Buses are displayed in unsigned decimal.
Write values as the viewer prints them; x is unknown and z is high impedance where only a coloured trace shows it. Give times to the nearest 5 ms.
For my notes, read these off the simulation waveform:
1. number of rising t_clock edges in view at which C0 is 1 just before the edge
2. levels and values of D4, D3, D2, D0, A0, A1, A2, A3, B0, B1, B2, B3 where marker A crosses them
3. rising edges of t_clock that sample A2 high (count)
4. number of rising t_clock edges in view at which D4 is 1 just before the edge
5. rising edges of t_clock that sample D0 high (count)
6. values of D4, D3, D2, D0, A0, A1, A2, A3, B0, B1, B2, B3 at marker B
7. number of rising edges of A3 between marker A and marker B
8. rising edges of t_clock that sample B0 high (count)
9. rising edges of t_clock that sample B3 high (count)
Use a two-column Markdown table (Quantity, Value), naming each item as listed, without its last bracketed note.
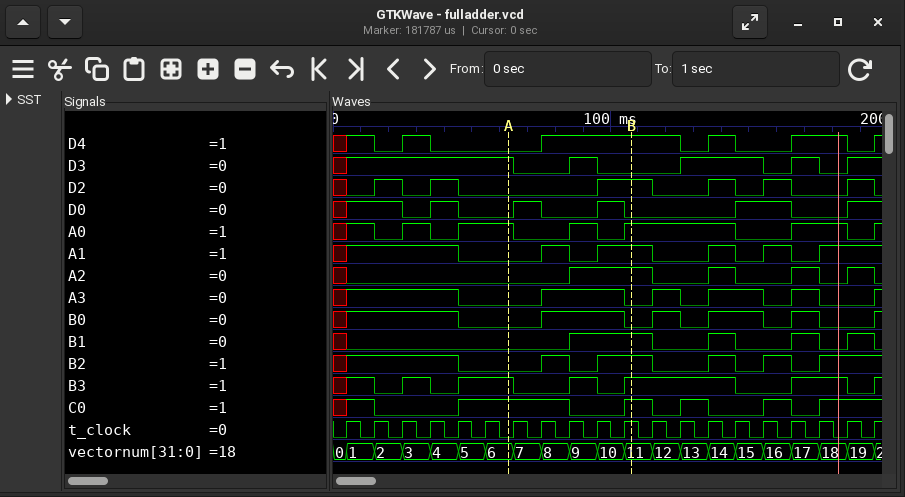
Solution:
| Quantity | Value |
|---|---|
| number of rising t_clock edges in view at which C0 is 1 just before the edge | 10 |
| levels and values of D4, D3, D2, D0, A0, A1, A2, A3, B0, B1, B2, B3 where marker A crosses them | D4=0, D3=1, D2=0, D0=0, A0=1, A1=0, A2=0, A3=0, B0=0, B1=0, B2=0, B3=1 |
| rising edges of t_clock that sample A2 high | 6 |
| number of rising t_clock edges in view at which D4 is 1 just before the edge | 10 |
| rising edges of t_clock that sample D0 high | 8 |
| values of D4, D3, D2, D0, A0, A1, A2, A3, B0, B1, B2, B3 at marker B | D4=1, D3=0, D2=1, D0=0, A0=1, A1=1, A2=1, A3=0, B0=0, B1=1, B2=1, B3=1 |
| number of rising edges of A3 between marker A and marker B | 1 |
| rising edges of t_clock that sample B0 high | 11 |
| rising edges of t_clock that sample B3 high | 11 |
